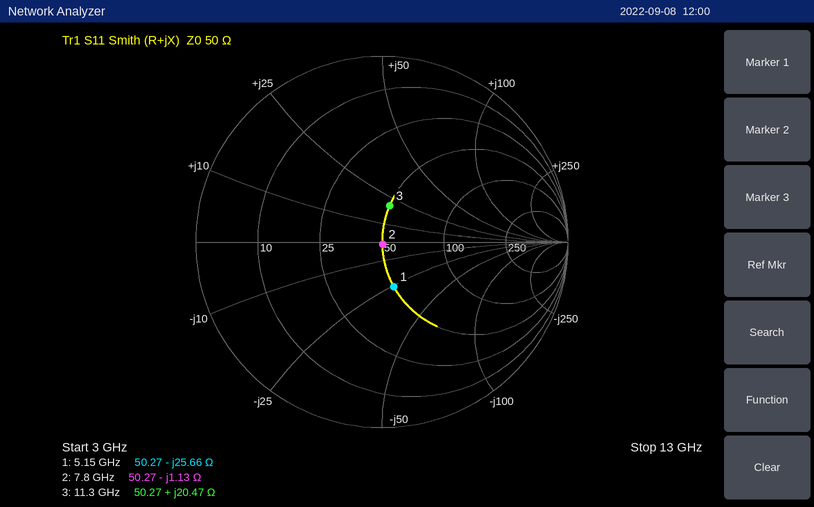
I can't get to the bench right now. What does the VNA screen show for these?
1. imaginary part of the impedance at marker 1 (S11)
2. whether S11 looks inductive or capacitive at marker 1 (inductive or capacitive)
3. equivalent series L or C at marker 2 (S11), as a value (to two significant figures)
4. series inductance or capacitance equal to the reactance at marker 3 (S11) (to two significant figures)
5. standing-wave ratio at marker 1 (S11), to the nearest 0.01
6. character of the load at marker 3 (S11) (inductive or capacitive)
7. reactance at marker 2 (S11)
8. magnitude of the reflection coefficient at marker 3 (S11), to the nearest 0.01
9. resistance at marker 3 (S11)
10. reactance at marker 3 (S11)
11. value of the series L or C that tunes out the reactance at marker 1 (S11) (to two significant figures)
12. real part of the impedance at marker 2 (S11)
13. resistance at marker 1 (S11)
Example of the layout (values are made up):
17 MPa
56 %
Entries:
-25.66 Ω
capacitive
18 pF
290 pH
1.66
inductive
-1.13 Ω
0.20
50.27 Ω
+20.47 Ω
790 pH
50.27 Ω
50.27 Ω
